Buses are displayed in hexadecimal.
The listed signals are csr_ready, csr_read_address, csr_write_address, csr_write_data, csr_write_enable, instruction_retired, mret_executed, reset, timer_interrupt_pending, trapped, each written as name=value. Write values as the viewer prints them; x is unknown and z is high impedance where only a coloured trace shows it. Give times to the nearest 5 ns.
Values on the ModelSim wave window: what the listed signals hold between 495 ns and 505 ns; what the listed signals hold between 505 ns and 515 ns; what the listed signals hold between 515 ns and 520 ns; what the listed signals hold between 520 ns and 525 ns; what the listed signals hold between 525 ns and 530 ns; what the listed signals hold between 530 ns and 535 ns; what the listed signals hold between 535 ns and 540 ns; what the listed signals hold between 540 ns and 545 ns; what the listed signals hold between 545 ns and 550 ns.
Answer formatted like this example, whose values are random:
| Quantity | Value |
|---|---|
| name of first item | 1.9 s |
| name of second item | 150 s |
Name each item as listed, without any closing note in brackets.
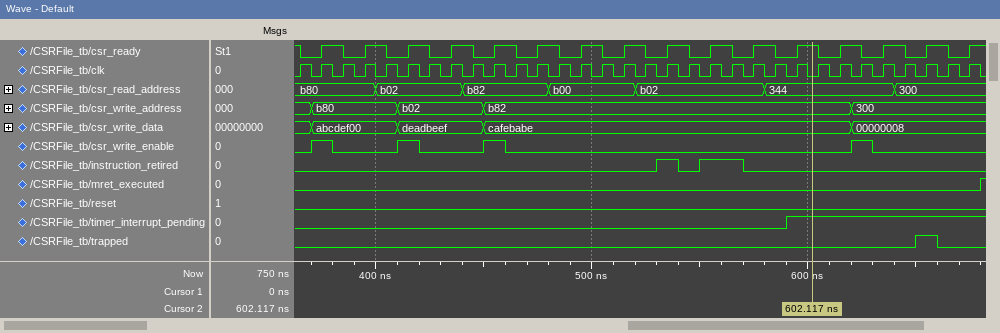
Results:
| Quantity | Value |
|---|---|
| what the listed signals hold between 495 ns and 505 ns | csr_ready=1, csr_read_address=b00, csr_write_address=b82, csr_write_data=cafebabe, csr_write_enable=0, instruction_retired=0, mret_executed=0, reset=0, timer_interrupt_pending=0, trapped=0 |
| what the listed signals hold between 505 ns and 515 ns | csr_ready=0, csr_read_address=b00, csr_write_address=b82, csr_write_data=cafebabe, csr_write_enable=0, instruction_retired=0, mret_executed=0, reset=0, timer_interrupt_pending=0, trapped=0 |
| what the listed signals hold between 515 ns and 520 ns | csr_ready=1, csr_read_address=b00, csr_write_address=b82, csr_write_data=cafebabe, csr_write_enable=0, instruction_retired=0, mret_executed=0, reset=0, timer_interrupt_pending=0, trapped=0 |
| what the listed signals hold between 520 ns and 525 ns | csr_ready=1, csr_read_address=b02, csr_write_address=b82, csr_write_data=cafebabe, csr_write_enable=0, instruction_retired=0, mret_executed=0, reset=0, timer_interrupt_pending=0, trapped=0 |
| what the listed signals hold between 525 ns and 530 ns | csr_ready=0, csr_read_address=b02, csr_write_address=b82, csr_write_data=cafebabe, csr_write_enable=0, instruction_retired=0, mret_executed=0, reset=0, timer_interrupt_pending=0, trapped=0 |
| what the listed signals hold between 530 ns and 535 ns | csr_ready=0, csr_read_address=b02, csr_write_address=b82, csr_write_data=cafebabe, csr_write_enable=0, instruction_retired=1, mret_executed=0, reset=0, timer_interrupt_pending=0, trapped=0 |
| what the listed signals hold between 535 ns and 540 ns | csr_ready=1, csr_read_address=b02, csr_write_address=b82, csr_write_data=cafebabe, csr_write_enable=0, instruction_retired=1, mret_executed=0, reset=0, timer_interrupt_pending=0, trapped=0 |
| what the listed signals hold between 540 ns and 545 ns | csr_ready=1, csr_read_address=b02, csr_write_address=b82, csr_write_data=cafebabe, csr_write_enable=0, instruction_retired=0, mret_executed=0, reset=0, timer_interrupt_pending=0, trapped=0 |
| what the listed signals hold between 545 ns and 550 ns | csr_ready=0, csr_read_address=b02, csr_write_address=b82, csr_write_data=cafebabe, csr_write_enable=0, instruction_retired=0, mret_executed=0, reset=0, timer_interrupt_pending=0, trapped=0 |
